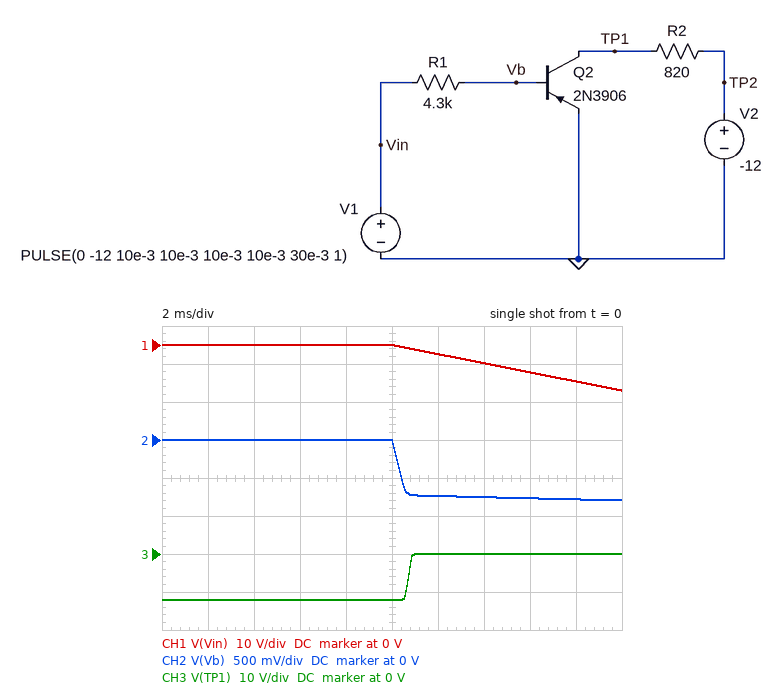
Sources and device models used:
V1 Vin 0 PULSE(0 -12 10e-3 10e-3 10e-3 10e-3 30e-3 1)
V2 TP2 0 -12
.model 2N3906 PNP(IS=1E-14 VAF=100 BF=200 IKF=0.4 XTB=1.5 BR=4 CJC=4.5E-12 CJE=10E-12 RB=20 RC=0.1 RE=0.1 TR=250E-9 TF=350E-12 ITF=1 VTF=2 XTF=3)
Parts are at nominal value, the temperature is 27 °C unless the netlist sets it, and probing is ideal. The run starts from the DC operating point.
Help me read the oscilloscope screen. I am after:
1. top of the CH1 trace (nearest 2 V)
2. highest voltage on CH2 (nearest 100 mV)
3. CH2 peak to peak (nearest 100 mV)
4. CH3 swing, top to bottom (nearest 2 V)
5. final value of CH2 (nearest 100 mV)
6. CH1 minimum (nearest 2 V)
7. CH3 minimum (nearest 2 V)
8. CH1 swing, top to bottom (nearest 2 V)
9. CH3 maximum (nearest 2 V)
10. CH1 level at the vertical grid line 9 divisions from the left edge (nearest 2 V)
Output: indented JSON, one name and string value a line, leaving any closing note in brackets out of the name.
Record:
{
  "top of the CH1 trace": "0 V",
  "highest voltage on CH2": "0 V",
  "CH2 peak to peak": "800 mV",
  "CH3 swing, top to bottom": "12 V",
  "final value of CH2": "-800 mV",
  "CH1 minimum": "-12 V",
  "CH3 minimum": "-12 V",
  "CH1 swing, top to bottom": "12 V",
  "CH3 maximum": "0 V",
  "CH1 level at the vertical grid line 9 divisions from the left edge": "-10 V"
}
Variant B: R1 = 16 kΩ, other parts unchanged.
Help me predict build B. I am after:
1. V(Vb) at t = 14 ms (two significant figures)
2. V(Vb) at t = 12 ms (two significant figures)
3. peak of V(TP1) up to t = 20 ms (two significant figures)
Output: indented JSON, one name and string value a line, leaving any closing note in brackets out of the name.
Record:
{
  "V(Vb) at t = 14 ms": "-730 mV",
  "V(Vb) at t = 12 ms": "-730 mV",
  "peak of V(TP1) up to t = 20 ms": "-55 mV"
}
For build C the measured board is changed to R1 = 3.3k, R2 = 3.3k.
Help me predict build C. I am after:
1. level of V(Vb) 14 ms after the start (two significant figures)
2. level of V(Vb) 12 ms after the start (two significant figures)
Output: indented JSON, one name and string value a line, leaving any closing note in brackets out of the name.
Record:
{
  "level of V(Vb) 14 ms after the start": "-740 mV",
  "level of V(Vb) 12 ms after the start": "-710 mV"
}
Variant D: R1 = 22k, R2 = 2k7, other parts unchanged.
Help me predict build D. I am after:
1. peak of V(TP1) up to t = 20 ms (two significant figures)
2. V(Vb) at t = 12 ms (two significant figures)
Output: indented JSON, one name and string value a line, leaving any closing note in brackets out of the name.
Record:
{
  "peak of V(TP1) up to t = 20 ms": "-34 mV",
  "V(Vb) at t = 12 ms": "-700 mV"
}
